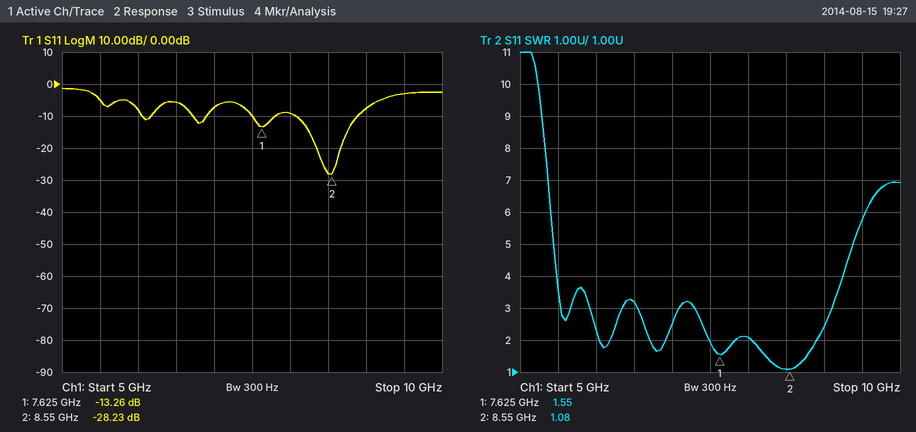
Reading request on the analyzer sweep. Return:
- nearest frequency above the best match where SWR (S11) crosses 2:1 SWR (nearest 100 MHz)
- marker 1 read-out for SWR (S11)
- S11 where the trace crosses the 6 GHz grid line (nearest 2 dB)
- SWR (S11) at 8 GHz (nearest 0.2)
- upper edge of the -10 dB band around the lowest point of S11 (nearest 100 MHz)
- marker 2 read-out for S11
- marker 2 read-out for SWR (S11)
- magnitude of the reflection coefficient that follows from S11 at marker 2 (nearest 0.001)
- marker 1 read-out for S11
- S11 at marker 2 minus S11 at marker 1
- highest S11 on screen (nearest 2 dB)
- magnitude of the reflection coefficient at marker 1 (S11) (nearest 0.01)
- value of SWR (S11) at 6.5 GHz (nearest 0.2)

8.9 GHz
1.55
-8 dB
2.0
8.9 GHz
-28.23 dB
1.08
0.039
-13.26 dB
-14.97 dB
-2 dB
0.22
3.2
